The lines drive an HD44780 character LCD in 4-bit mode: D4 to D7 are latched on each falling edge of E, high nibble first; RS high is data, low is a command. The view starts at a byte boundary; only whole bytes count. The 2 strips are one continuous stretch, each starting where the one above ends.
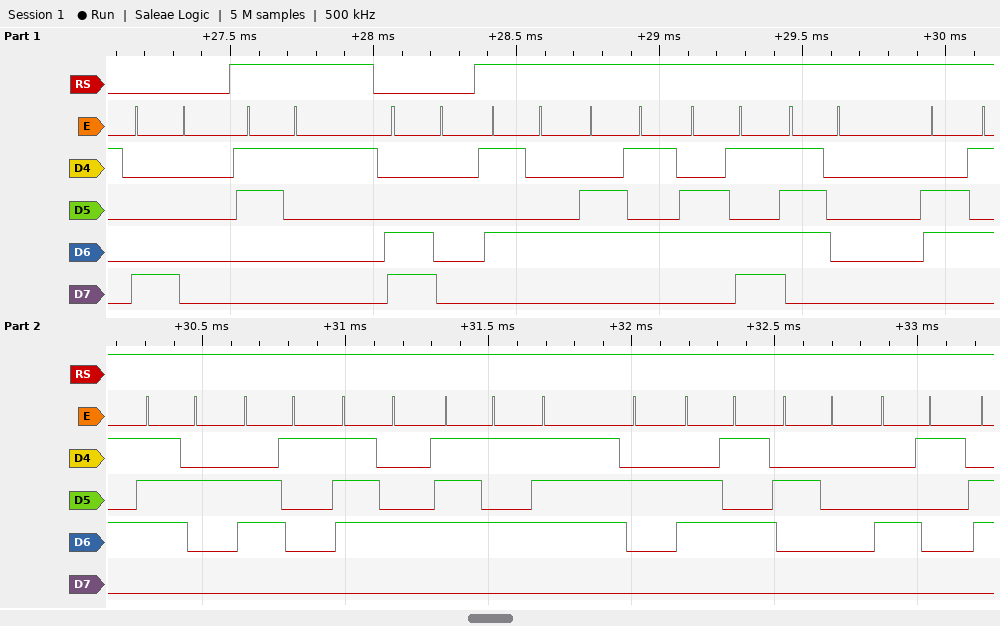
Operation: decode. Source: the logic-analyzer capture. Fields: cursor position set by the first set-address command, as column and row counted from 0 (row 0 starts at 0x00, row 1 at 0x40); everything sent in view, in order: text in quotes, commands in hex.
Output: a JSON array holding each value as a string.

["column 0, row 0", "0x80 \"1\" 0xC0 \"Temperature A\""]
